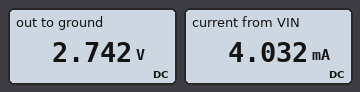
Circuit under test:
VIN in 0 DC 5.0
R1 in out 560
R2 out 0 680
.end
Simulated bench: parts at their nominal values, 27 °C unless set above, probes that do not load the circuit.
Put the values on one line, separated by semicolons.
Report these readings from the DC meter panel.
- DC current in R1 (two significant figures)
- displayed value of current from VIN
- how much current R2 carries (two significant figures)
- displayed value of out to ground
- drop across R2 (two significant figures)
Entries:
4.0 mA; 4.032 mA; 4.0 mA; 2.742 V; 2.7 V
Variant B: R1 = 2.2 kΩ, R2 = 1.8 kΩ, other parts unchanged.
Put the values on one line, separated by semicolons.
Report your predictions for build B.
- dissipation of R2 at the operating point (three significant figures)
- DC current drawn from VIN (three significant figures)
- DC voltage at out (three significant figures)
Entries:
2.81 mW; 1.25 mA; 2.25 V
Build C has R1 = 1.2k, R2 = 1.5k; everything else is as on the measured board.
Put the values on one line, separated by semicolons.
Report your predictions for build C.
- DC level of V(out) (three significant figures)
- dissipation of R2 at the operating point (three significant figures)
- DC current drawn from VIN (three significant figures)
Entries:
2.78 V; 5.14 mW; 1.85 mA
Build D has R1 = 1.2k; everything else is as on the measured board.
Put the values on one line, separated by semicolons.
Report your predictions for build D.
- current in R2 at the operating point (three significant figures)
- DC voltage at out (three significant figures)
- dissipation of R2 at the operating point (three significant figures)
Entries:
2.66 mA; 1.81 V; 4.81 mW
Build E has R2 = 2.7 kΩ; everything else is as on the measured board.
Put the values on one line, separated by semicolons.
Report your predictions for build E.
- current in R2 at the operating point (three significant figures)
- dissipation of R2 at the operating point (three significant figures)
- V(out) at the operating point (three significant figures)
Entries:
1.53 mA; 6.35 mW; 4.14 V
